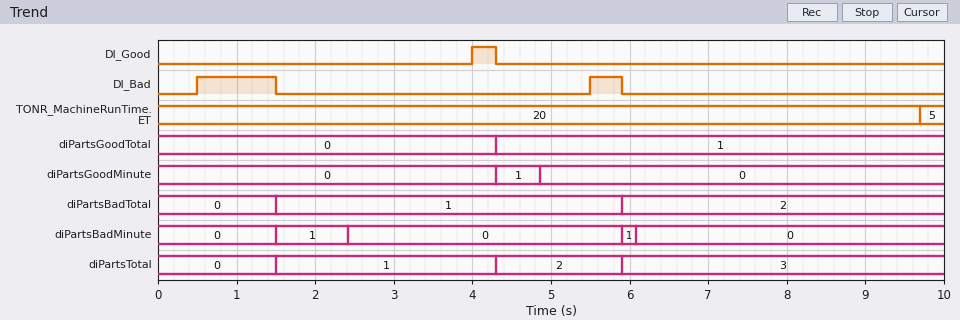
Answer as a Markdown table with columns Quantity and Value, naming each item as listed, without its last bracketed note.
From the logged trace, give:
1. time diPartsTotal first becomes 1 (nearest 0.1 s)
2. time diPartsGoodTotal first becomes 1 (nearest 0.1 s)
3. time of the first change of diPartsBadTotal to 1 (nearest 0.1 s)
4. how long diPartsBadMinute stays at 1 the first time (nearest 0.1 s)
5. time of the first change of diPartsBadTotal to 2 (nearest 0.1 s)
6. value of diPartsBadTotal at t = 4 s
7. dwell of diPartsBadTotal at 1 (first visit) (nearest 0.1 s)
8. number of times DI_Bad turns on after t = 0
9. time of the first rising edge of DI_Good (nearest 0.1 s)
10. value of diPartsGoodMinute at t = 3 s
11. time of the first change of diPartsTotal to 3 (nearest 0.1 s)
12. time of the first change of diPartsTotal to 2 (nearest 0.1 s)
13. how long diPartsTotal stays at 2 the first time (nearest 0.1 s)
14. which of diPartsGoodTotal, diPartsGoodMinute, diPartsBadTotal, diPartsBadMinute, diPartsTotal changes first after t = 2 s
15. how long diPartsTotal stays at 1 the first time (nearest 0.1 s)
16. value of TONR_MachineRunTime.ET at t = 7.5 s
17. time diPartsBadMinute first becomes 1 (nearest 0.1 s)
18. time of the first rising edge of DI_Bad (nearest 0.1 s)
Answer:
| Quantity | Value |
|---|---|
| time diPartsTotal first becomes 1 | 1.5 s |
| time diPartsGoodTotal first becomes 1 | 4.3 s |
| time of the first change of diPartsBadTotal to 1 | 1.5 s |
| how long diPartsBadMinute stays at 1 the first time | 0.9 s |
| time of the first change of diPartsBadTotal to 2 | 5.9 s |
| value of diPartsBadTotal at t = 4 s | 1 |
| dwell of diPartsBadTotal at 1 (first visit) | 4.4 s |
| number of times DI_Bad turns on after t = 0 | 2 |
| time of the first rising edge of DI_Good | 4.0 s |
| value of diPartsGoodMinute at t = 3 s | 0 |
| time of the first change of diPartsTotal to 3 | 5.9 s |
| time of the first change of diPartsTotal to 2 | 4.3 s |
| how long diPartsTotal stays at 2 the first time | 1.6 s |
| which of diPartsGoodTotal, diPartsGoodMinute, diPartsBadTotal, diPartsBadMinute, diPartsTotal changes first after t = 2 s | diPartsBadMinute |
| how long diPartsTotal stays at 1 the first time | 2.8 s |
| value of TONR_MachineRunTime.ET at t = 7.5 s | 20 |
| time diPartsBadMinute first becomes 1 | 1.5 s |
| time of the first rising edge of DI_Bad | 0.5 s |
